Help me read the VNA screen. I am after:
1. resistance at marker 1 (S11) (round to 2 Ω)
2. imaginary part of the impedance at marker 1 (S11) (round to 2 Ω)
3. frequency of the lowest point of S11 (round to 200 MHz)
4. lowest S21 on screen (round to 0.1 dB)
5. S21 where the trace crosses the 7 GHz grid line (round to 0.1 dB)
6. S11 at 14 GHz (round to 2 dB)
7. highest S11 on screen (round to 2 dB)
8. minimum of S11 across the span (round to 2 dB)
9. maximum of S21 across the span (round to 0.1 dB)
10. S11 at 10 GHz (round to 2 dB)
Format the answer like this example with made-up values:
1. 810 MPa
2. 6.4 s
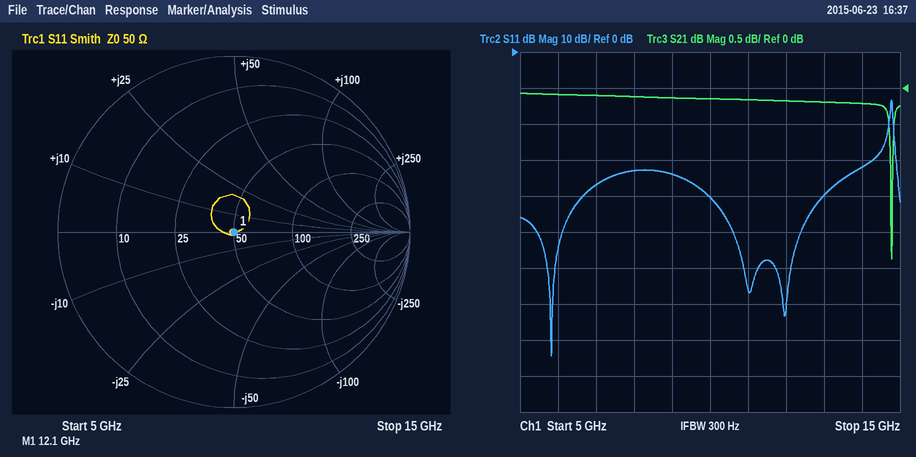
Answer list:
1. 50 Ω
2. 0 Ω
3. 5.8 GHz
4. -2.4 dB
5. -0.1 dB
6. -32 dB
7. -14 dB
8. -84 dB
9. -0.1 dB
10. -40 dB
